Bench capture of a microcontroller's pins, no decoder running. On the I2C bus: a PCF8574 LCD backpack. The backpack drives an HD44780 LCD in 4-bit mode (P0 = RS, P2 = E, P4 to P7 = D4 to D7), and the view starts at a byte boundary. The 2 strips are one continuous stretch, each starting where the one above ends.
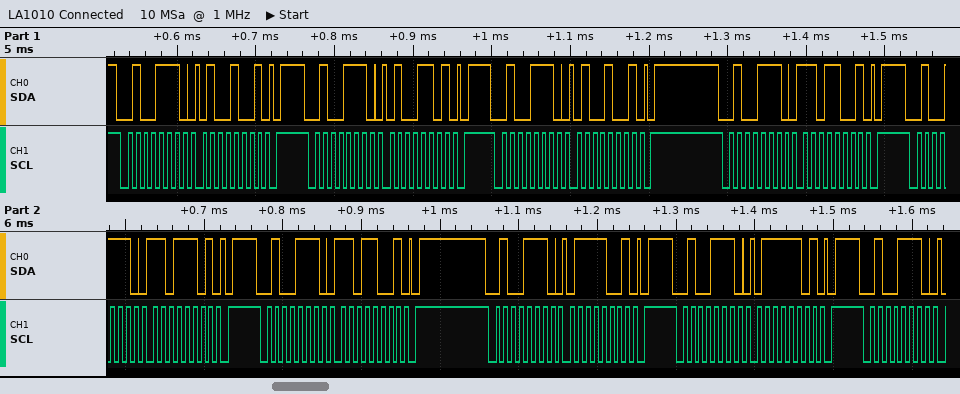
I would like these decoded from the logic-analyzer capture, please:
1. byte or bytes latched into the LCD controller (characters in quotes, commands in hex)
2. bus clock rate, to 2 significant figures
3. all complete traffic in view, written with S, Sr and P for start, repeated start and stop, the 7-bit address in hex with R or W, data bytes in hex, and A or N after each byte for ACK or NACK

'M'
100 kHz
S 27W A 49 A P S 27W A 4D A P S 27W A 49 A P S 27W A D9 A P S 27W A DD A P S 27W A D9 A P S 27W A 79 A P S 27W A 7D A P S 27W A
